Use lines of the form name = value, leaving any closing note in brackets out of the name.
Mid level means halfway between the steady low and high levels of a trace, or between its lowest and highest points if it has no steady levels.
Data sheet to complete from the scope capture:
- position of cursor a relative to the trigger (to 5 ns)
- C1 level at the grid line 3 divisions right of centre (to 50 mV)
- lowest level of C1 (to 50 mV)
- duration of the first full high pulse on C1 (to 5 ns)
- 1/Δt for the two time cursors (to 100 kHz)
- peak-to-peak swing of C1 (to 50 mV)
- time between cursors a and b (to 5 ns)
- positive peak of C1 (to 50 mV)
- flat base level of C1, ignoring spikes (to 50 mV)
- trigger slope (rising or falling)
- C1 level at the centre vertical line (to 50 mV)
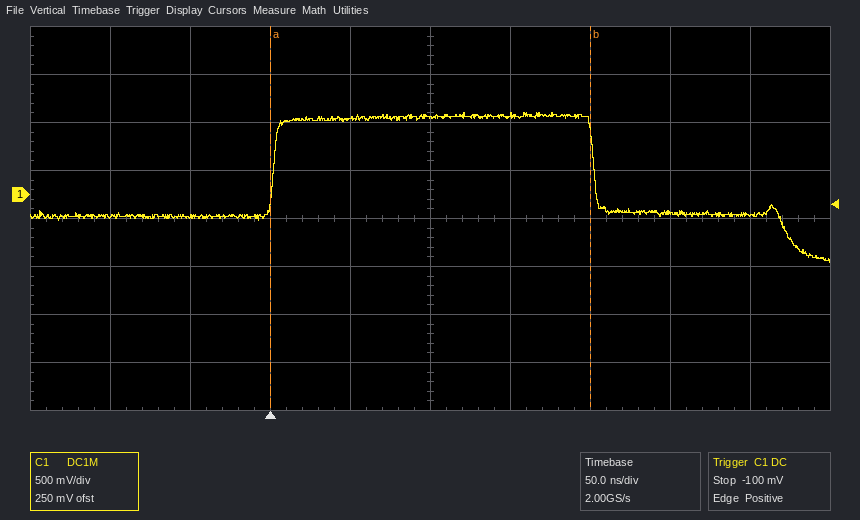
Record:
position of cursor a relative to the trigger = 0 ns
C1 level at the grid line 3 divisions right of centre = -200 mV
lowest level of C1 = -700 mV
duration of the first full high pulse on C1 = 200 ns
1/Δt for the two time cursors = 5.0 MHz
peak-to-peak swing of C1 = 1.55 V
time between cursors a and b = 200 ns
positive peak of C1 = 850 mV
flat base level of C1, ignoring spikes = -200 mV
trigger slope = rising
C1 level at the centre vertical line = 800 mV
